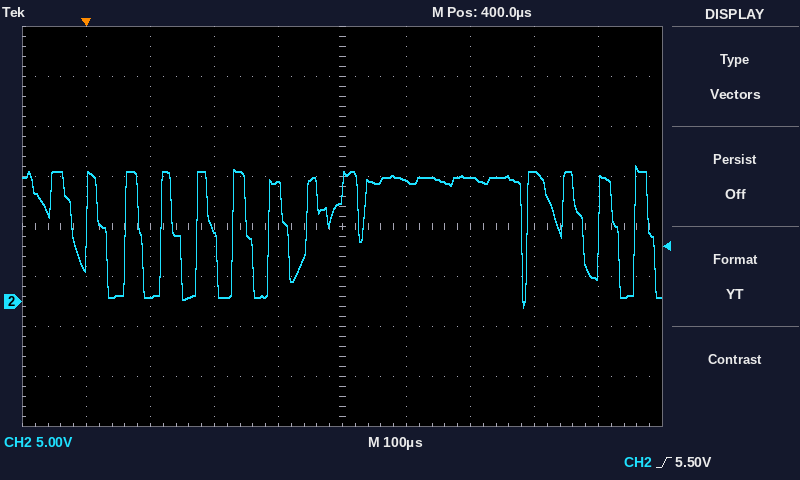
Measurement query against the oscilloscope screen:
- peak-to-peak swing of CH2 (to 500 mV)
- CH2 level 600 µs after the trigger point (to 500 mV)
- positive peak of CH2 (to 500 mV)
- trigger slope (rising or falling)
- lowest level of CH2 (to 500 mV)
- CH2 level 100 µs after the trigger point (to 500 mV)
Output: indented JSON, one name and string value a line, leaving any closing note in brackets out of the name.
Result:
{
  "peak-to-peak swing of CH2": "14.0 V",
  "CH2 level 600 µs after the trigger point": "12.5 V",
  "positive peak of CH2": "13.5 V",
  "trigger slope": "rising",
  "lowest level of CH2": "-500 mV",
  "CH2 level 100 µs after the trigger point": "500 mV"
}
